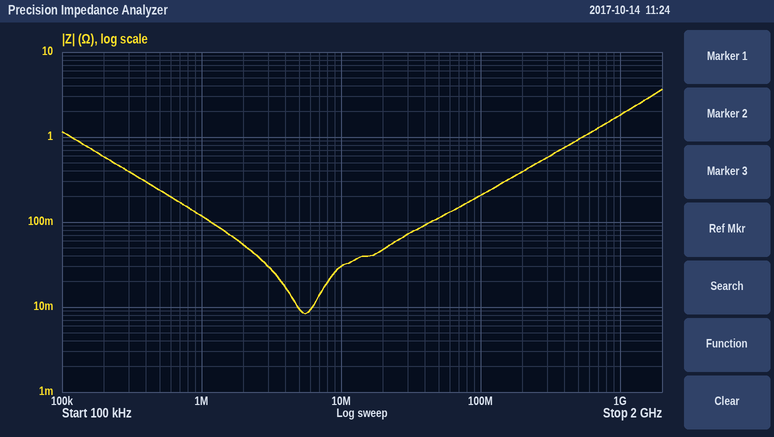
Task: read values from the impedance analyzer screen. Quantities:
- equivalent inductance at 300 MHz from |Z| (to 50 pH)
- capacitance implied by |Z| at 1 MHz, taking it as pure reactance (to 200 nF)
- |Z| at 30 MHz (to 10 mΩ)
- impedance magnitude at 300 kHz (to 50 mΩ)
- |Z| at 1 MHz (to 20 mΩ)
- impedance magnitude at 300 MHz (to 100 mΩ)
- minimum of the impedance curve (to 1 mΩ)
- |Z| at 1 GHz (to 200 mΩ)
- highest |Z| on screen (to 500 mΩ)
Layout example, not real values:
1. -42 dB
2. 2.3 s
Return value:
1. 300 pH
2. 1.4 µF
3. 70 mΩ
4. 400 mΩ
5. 120 mΩ
6. 600 mΩ
7. 8 mΩ
8. 1.8 Ω
9. 3.5 Ω
